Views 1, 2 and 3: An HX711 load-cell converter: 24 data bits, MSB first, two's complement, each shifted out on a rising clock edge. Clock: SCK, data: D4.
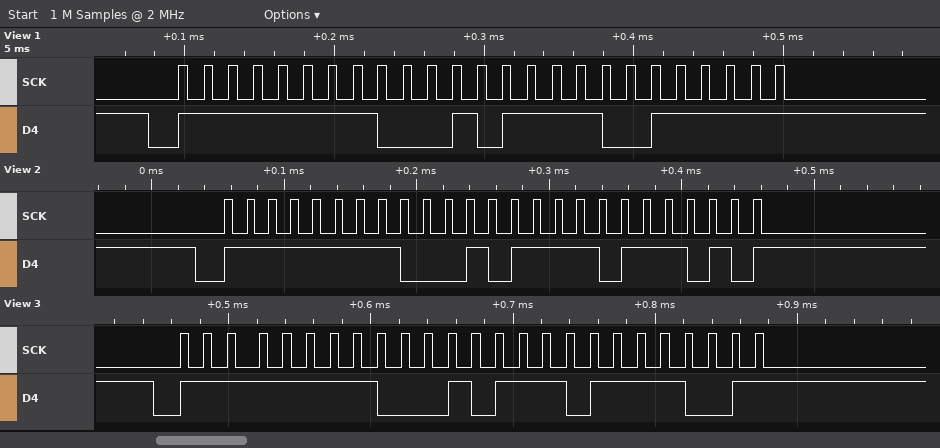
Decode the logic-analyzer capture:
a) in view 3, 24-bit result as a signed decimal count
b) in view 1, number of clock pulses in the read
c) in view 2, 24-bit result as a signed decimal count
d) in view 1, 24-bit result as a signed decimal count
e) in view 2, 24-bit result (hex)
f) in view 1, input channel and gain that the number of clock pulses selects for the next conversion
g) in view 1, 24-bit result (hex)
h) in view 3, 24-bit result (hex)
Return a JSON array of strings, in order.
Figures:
["-59527", "25", "-59462", "-59489", "0xFF17BA", "channel A, gain 128", "0xFF179F", "0xFF1779"]
